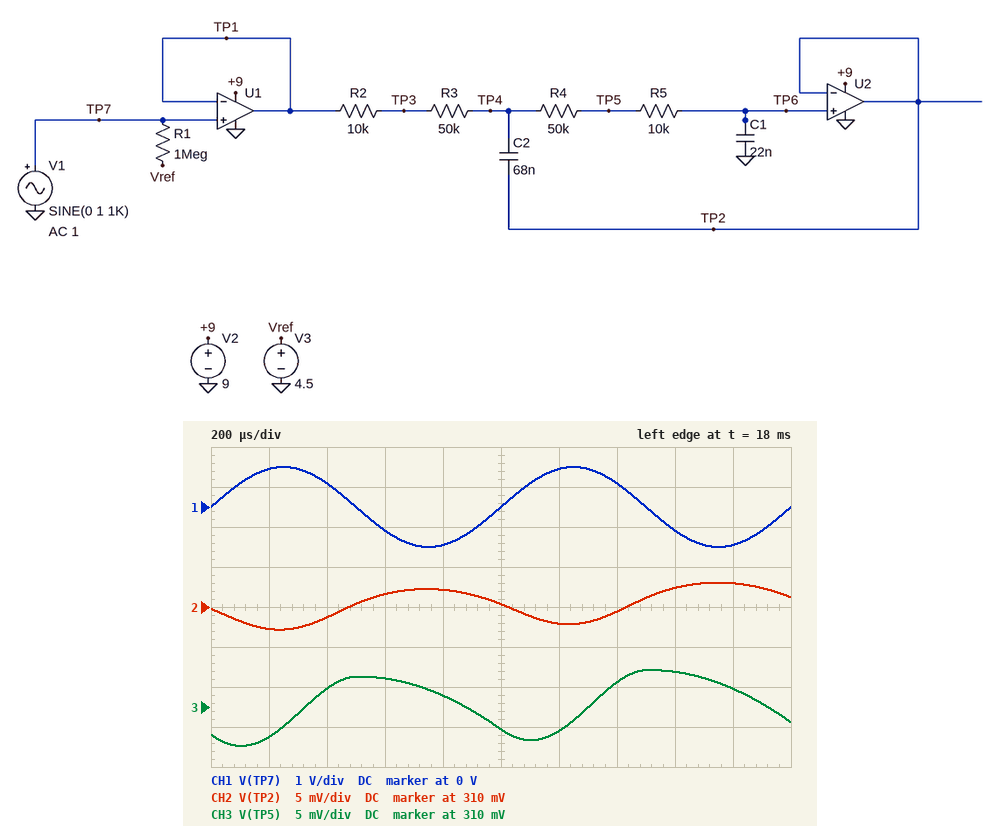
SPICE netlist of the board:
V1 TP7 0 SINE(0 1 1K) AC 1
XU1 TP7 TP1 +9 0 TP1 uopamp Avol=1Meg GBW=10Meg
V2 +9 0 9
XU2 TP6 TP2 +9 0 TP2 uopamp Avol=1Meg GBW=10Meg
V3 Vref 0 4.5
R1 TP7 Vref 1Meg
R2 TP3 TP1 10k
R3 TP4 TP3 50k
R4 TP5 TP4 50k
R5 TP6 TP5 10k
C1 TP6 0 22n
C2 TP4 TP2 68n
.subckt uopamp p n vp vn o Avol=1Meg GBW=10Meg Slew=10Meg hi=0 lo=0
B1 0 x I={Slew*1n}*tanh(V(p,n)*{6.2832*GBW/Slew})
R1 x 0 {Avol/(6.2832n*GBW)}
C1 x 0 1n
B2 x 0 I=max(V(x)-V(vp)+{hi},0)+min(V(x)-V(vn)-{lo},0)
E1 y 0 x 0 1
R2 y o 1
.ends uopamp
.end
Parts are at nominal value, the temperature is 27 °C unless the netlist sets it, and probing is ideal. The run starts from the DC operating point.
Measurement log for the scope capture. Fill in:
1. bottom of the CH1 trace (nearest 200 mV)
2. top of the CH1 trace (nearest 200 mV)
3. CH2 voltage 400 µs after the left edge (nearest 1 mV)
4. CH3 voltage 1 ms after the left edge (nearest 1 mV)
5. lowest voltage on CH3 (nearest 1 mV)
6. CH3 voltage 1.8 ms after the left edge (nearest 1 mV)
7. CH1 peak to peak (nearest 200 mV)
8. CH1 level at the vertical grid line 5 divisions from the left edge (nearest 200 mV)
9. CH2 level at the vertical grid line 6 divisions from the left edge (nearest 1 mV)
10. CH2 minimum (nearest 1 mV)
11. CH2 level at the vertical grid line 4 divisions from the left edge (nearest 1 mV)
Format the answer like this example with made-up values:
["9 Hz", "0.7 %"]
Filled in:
["-1.0 V", "1.0 V", "309 mV", "307 mV", "305 mV", "312 mV", "2.0 V", "0 V", "308 mV", "307 mV", "312 mV"]
